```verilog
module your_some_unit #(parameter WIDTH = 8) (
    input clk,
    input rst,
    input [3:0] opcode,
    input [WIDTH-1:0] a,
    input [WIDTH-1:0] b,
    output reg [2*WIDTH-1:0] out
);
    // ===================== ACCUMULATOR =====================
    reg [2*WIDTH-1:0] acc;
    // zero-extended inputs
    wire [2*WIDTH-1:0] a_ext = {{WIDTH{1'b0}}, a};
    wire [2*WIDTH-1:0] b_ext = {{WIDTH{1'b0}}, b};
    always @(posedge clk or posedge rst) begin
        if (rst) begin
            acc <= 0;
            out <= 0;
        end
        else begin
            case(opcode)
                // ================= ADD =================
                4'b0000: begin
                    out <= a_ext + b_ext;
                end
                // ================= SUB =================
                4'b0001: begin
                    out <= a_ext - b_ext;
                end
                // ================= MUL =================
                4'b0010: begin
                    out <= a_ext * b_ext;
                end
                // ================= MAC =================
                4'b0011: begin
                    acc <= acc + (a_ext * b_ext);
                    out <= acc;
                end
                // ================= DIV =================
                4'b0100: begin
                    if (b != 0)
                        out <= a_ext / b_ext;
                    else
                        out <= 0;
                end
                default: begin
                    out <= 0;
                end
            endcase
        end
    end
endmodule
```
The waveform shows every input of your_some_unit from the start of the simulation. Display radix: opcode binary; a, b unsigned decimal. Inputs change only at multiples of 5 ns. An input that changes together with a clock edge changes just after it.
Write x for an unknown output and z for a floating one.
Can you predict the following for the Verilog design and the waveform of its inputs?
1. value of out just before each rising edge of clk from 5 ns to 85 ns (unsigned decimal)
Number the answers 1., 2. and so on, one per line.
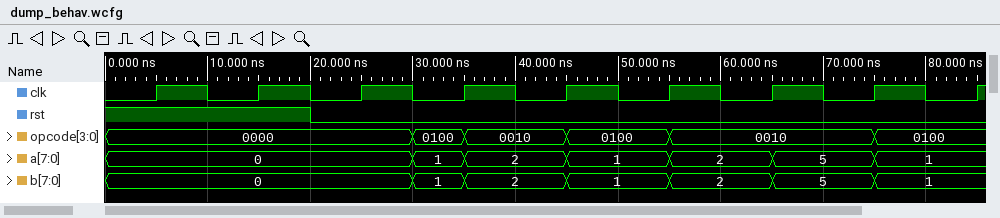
1. 0, 0, 0, 0, 1, 4, 1, 4, 25
